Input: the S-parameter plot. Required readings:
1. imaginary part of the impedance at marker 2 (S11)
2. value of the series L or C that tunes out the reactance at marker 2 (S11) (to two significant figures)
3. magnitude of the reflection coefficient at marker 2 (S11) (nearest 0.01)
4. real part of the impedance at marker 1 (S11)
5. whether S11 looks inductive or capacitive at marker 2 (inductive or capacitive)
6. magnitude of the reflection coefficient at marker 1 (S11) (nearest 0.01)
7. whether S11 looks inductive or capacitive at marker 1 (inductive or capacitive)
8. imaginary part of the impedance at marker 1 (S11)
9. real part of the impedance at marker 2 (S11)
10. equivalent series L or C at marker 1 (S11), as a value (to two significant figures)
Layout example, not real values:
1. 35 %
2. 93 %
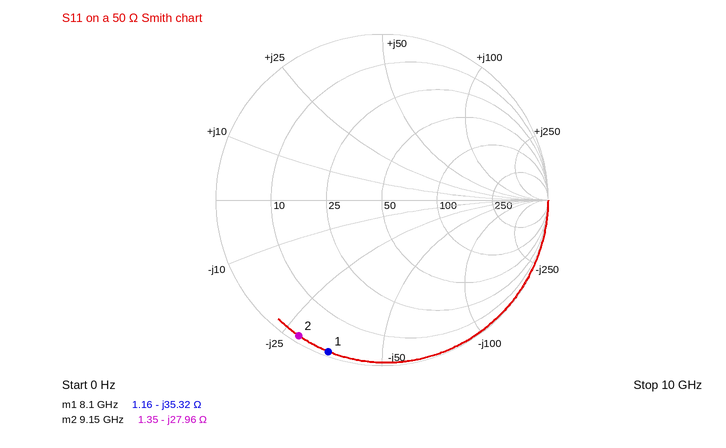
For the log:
1. -27.96 Ω
2. 490 pH
3. 0.96
4. 1.16 Ω
5. capacitive
6. 0.97
7. capacitive
8. -35.32 Ω
9. 1.35 Ω
10. 560 fF
